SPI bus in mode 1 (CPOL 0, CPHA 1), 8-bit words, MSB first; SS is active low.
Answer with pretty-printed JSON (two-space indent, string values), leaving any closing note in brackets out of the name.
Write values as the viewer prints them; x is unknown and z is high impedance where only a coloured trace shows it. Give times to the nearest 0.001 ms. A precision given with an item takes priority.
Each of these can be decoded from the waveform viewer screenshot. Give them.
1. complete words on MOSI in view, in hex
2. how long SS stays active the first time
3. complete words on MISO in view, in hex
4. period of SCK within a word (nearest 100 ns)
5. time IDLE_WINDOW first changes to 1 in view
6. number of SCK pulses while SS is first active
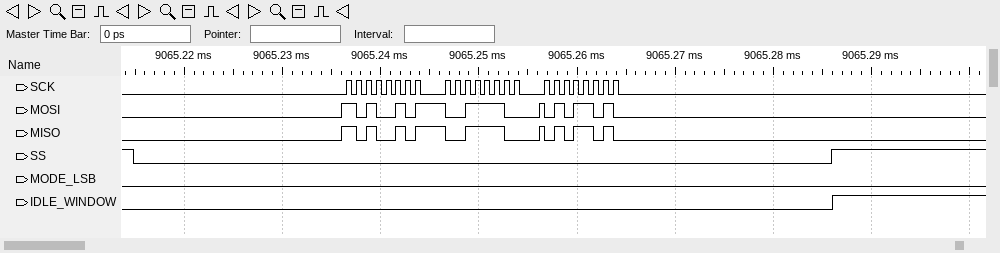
{
  "complete words on MOSI in view, in hex": "A5, 3C, 5A",
  "how long SS stays active the first time": "0.071 ms",
  "complete words on MISO in view, in hex": "A5, 3C, 5A",
  "period of SCK within a word": "1000 ns",
  "time IDLE_WINDOW first changes to 1 in view": "9065.286 ms",
  "number of SCK pulses while SS is first active": "24"
}
